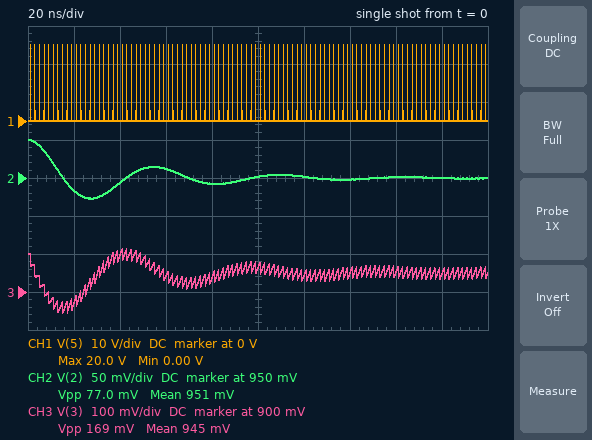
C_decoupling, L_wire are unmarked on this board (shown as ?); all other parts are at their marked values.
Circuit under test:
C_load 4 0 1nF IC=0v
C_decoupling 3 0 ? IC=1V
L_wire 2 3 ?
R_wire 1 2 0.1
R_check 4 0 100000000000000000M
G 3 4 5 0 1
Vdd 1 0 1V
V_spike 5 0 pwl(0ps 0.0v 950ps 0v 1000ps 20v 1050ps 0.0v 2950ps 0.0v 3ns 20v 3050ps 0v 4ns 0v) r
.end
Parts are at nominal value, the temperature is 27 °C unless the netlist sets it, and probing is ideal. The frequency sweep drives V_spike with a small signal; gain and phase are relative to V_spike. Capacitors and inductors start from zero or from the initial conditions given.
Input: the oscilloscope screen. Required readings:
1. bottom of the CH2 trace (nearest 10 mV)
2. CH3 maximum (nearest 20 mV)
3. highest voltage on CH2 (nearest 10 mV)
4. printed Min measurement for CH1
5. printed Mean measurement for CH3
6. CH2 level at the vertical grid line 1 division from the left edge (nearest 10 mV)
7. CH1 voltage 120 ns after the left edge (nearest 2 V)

920 mV
1.02 V
1.00 V
0.00 V
945 mV
930 mV
0 V
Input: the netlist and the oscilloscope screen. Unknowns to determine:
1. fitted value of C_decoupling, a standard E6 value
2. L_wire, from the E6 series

33 nF
2.2 nH
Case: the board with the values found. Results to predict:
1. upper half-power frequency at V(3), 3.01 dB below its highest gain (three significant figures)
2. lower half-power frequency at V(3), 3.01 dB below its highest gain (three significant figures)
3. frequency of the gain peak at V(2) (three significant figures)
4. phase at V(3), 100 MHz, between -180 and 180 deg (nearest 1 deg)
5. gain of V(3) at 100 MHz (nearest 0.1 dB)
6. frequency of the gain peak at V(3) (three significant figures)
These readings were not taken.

22.5 MHz
15.2 MHz
18.0 MHz
90 deg
-26.0 dB
18.6 MHz
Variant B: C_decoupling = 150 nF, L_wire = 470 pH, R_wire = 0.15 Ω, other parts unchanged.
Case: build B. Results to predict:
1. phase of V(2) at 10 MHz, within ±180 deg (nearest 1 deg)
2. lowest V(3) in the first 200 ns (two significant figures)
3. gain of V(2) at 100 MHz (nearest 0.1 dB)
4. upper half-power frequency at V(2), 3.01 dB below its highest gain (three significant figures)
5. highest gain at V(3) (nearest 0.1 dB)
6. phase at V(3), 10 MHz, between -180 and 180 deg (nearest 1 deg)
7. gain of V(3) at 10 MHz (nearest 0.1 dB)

117 deg
920 mV
-46.1 dB
8.18 MHz
-16.5 dB
128 deg
-20.3 dB
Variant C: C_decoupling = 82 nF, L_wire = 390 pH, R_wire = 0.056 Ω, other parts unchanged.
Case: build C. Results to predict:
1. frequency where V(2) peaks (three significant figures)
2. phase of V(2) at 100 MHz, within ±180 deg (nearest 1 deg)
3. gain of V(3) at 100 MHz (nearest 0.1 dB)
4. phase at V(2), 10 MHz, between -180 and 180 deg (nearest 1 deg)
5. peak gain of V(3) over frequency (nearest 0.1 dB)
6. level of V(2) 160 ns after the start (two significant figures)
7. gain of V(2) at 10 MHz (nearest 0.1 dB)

23.0 MHz
14 deg
-33.6 dB
162 deg
-19.1 dB
970 mV
-24.3 dB
